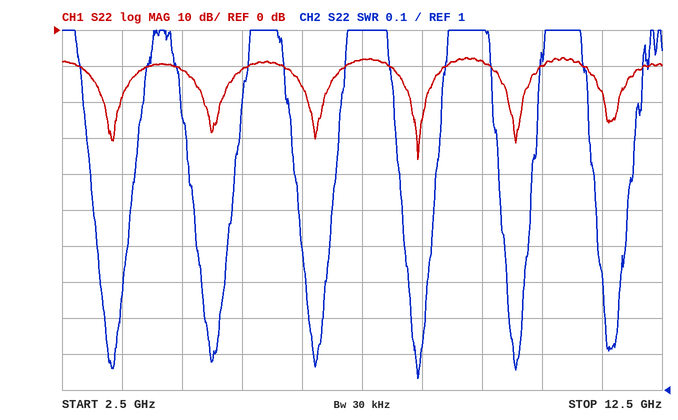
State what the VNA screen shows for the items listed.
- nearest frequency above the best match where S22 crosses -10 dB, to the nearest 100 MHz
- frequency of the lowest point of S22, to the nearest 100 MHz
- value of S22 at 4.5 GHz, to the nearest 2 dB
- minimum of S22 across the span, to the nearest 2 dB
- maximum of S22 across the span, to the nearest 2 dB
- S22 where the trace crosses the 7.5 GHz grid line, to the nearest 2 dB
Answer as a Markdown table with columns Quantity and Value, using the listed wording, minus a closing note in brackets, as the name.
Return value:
| Quantity | Value |
|---|---|
| nearest frequency above the best match where S22 crosses -10 dB, to the nearest 100 MHz | 8.9 GHz |
| frequency of the lowest point of S22, to the nearest 100 MHz | 8.4 GHz |
| value of S22 at 4.5 GHz, to the nearest 2 dB | -12 dB |
| minimum of S22 across the span, to the nearest 2 dB | -36 dB |
| maximum of S22 across the span, to the nearest 2 dB | -8 dB |
| S22 where the trace crosses the 7.5 GHz grid line, to the nearest 2 dB | -8 dB |
